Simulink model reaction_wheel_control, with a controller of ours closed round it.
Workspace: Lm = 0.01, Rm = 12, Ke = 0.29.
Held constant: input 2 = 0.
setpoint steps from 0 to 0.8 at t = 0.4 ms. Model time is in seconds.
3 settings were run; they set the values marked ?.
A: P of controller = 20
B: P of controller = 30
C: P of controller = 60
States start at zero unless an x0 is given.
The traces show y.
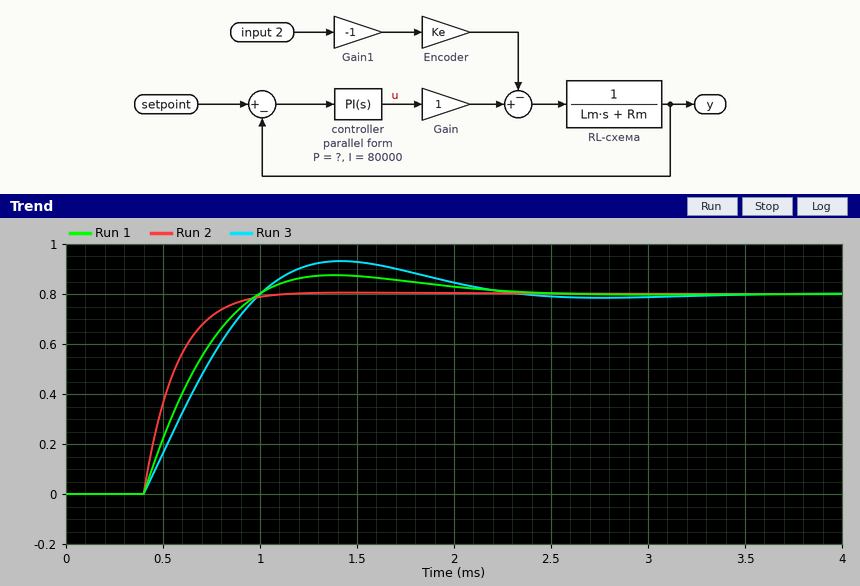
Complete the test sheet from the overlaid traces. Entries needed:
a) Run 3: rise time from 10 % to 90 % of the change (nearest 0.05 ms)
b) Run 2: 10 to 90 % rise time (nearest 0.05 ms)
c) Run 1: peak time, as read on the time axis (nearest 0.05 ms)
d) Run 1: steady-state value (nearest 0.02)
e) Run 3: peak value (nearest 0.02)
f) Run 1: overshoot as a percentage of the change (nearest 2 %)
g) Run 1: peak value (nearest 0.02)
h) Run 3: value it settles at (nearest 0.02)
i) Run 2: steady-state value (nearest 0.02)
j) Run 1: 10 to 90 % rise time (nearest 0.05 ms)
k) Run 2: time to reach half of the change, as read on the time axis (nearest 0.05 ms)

0.45 ms
0.35 ms
1.40 ms
0.80
0.94
10 %
0.88
0.80
0.80
0.45 ms
0.50 ms
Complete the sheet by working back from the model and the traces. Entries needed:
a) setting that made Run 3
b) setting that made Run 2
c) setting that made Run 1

A
C
B
